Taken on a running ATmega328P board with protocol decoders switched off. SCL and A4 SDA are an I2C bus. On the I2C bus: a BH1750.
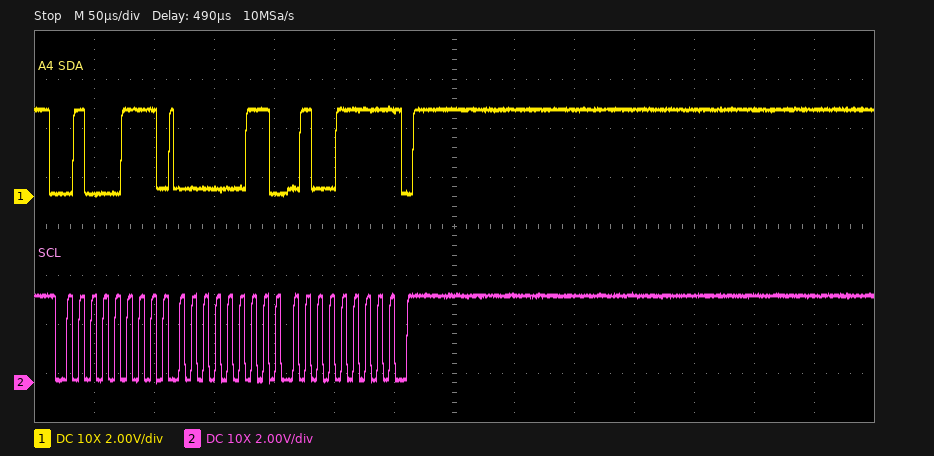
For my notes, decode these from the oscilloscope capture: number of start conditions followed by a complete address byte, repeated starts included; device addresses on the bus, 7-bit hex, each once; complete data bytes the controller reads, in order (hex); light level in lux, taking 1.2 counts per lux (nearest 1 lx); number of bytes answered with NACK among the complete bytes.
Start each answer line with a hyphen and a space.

- 1
- 0x23
- 03 4F
- 706 lx
- 1
